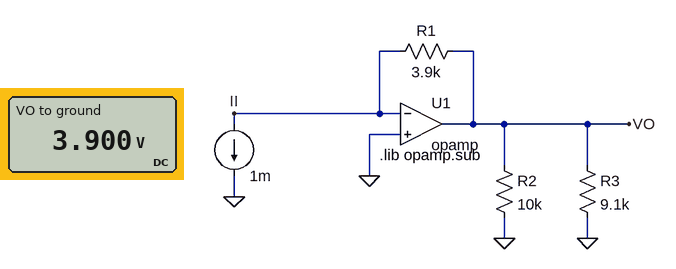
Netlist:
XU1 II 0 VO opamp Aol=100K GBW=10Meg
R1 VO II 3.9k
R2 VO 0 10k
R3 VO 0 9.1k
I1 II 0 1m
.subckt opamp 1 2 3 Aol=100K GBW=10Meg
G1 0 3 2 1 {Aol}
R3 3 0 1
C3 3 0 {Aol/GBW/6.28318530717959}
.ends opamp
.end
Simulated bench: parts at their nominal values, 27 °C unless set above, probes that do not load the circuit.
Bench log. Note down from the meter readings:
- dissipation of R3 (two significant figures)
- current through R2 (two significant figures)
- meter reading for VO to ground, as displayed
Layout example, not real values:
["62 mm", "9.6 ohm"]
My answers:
["1.7 mW", "390 µA", "3.900 V"]
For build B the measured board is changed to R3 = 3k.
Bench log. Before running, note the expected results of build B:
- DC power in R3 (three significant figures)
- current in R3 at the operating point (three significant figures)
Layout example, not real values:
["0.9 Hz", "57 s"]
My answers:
["5.07 mW", "1.30 mA"]
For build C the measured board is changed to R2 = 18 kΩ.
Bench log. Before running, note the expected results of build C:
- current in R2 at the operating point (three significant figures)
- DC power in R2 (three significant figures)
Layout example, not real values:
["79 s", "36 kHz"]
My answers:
["217 µA", "845 µW"]
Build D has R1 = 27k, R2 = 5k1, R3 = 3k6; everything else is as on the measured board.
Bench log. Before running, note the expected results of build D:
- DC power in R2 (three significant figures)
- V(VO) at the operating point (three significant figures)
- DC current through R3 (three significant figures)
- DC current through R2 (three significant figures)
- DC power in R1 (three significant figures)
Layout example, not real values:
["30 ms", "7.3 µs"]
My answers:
["143 mW", "27.0 V", "7.50 mA", "5.29 mA", "27.0 mW"]
